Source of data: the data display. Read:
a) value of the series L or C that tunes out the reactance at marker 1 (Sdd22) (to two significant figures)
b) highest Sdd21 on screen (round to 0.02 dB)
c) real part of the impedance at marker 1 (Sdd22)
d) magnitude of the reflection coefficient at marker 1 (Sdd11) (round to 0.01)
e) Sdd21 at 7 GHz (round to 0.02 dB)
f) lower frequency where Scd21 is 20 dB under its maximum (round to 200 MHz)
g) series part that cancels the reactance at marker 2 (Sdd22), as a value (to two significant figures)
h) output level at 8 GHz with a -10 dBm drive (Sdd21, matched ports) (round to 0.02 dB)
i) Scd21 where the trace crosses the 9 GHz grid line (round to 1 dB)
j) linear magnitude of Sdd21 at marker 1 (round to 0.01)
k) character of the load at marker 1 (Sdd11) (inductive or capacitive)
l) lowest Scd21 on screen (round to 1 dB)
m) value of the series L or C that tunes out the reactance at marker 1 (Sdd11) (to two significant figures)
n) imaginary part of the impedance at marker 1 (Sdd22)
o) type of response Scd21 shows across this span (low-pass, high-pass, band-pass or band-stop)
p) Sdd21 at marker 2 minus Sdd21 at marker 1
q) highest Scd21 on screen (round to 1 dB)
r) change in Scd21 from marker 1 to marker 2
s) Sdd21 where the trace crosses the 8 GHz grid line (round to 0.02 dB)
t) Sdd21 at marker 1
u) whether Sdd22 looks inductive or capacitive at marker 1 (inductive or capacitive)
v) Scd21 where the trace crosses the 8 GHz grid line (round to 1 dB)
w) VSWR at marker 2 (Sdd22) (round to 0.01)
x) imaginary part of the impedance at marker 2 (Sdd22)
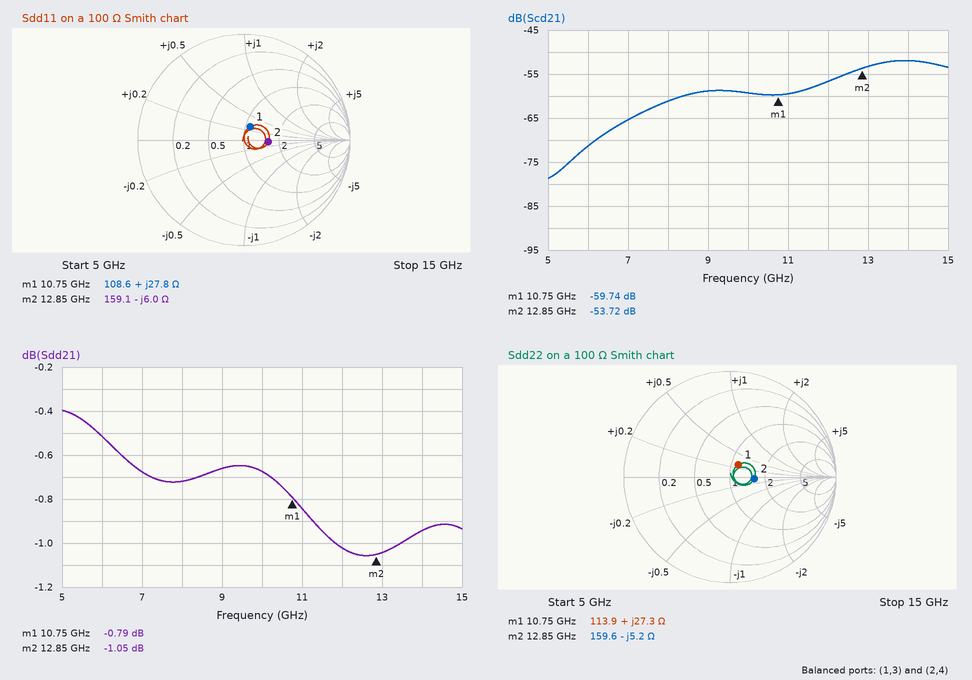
540 fF
-0.40 dB
113.9 Ω
0.14
-0.68 dB
6.0 GHz
64 pH
-10.72 dBm
-59 dB
0.91
inductive
-79 dB
530 fF
+27.3 Ω
high-pass
-0.26 dB
-52 dB
6.02 dB
-0.72 dB
-0.79 dB
inductive
-61 dB
1.60
-5.2 Ω
